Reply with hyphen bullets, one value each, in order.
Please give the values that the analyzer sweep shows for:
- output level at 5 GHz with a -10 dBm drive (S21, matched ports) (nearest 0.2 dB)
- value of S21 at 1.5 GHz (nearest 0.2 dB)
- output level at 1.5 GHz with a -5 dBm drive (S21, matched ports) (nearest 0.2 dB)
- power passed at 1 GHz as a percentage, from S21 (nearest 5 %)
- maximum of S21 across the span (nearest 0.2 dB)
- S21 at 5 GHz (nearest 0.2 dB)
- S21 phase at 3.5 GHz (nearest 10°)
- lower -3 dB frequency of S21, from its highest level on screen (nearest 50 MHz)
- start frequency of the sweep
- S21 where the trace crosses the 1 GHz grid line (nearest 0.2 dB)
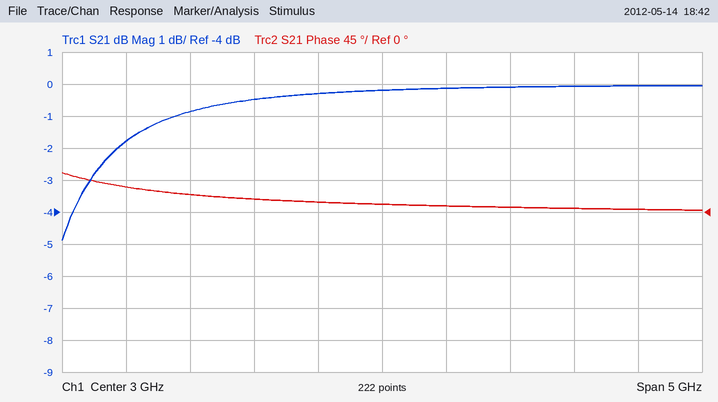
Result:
- -10.0 dBm
- -0.8 dB
- -5.8 dBm
- 65 %
- 0.0 dB
- 0.0 dB
- 10°
- 700 MHz
- 500 MHz
- -1.8 dB
